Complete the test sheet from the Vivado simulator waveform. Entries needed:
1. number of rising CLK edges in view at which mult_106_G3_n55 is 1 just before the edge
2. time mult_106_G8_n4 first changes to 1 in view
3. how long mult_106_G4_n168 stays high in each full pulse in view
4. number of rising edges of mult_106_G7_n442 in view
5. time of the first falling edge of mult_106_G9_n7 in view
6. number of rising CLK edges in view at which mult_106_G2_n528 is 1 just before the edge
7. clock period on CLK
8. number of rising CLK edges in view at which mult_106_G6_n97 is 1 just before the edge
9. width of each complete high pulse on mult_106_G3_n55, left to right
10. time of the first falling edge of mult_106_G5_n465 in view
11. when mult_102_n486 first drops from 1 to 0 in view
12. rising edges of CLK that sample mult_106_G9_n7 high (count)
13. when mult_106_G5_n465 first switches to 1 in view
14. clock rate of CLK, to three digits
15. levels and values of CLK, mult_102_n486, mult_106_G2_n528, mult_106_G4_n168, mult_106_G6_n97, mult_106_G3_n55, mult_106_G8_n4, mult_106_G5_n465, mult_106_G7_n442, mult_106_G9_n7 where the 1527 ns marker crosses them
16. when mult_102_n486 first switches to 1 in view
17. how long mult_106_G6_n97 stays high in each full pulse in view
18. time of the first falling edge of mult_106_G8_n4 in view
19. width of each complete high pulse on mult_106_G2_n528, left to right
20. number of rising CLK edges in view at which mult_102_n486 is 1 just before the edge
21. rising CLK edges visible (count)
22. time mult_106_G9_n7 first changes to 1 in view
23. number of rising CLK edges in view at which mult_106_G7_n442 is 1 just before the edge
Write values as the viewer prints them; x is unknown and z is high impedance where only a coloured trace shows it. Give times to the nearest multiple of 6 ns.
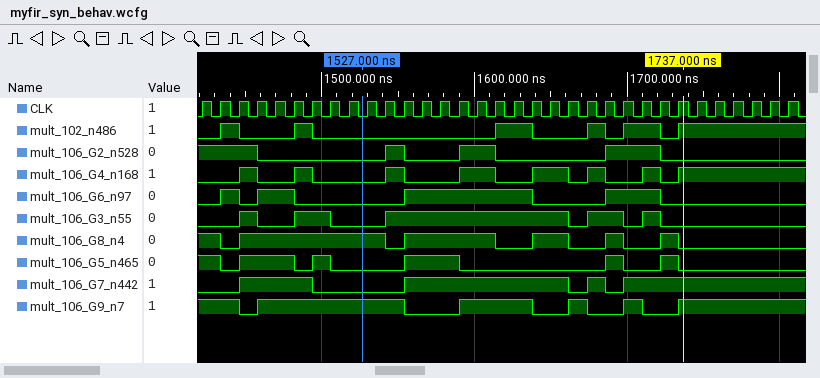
16
1446 ns
12 ns, 12 ns, 12 ns, 24 ns, 24 ns, 12 ns, 12 ns
4
1446 ns
10
12 ns
13
12 ns, 24 ns, 120 ns, 24 ns, 12 ns
1434 ns
1446 ns
23
1446 ns
83.3 MHz
CLK=0, mult_102_n486=0, mult_106_G2_n528=0, mult_106_G4_n168=0, mult_106_G6_n97=0, mult_106_G3_n55=0, mult_106_G8_n4=1, mult_106_G5_n465=0, mult_106_G7_n442=0, mult_106_G9_n7=1
1434 ns
12 ns, 24 ns, 84 ns, 36 ns
1434 ns
12 ns, 24 ns, 36 ns
13
33
1458 ns
23
